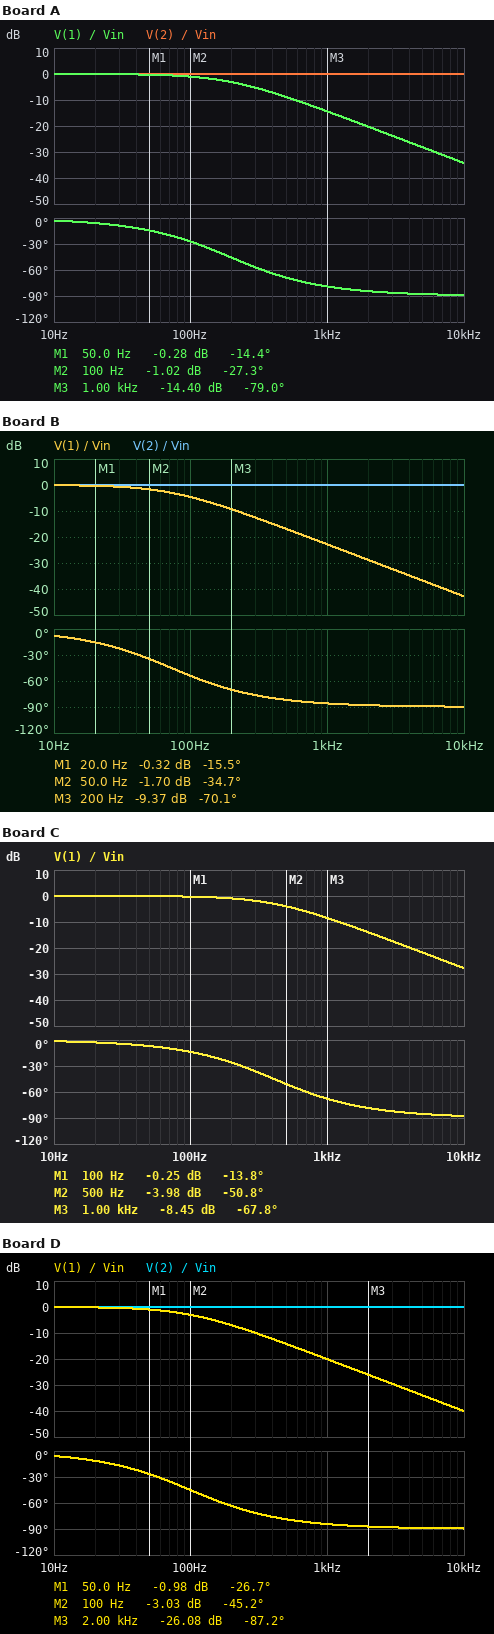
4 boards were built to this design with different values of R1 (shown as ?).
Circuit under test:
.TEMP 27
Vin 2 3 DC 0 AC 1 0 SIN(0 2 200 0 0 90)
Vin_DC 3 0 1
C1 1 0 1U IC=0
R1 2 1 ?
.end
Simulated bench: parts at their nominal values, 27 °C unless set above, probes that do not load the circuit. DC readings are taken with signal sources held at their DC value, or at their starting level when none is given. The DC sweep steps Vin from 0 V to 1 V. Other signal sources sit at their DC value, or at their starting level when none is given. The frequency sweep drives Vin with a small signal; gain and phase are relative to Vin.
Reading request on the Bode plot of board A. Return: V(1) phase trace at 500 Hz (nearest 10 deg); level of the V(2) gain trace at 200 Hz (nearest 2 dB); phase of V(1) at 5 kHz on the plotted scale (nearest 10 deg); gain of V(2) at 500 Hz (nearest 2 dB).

-70 deg
0 dB
-90 deg
0 dB
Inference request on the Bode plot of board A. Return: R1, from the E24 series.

820 Ω
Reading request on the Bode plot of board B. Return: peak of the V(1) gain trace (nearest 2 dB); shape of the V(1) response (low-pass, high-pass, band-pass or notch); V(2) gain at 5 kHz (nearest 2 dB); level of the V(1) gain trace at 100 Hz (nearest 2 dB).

0 dB
low-pass
0 dB
-4 dB
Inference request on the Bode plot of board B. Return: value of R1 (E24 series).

2.2 kΩ
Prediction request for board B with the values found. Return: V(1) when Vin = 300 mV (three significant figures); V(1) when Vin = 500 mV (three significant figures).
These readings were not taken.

1.30 V
1.50 V
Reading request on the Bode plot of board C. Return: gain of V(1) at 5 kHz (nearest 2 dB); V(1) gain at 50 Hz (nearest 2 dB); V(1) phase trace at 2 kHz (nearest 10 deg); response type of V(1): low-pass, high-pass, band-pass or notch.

-22 dB
0 dB
-80 deg
low-pass
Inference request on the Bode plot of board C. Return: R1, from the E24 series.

390 Ω
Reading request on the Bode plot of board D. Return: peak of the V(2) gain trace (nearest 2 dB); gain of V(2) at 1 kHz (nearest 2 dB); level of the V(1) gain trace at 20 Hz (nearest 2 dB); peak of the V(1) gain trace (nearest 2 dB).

0 dB
0 dB
0 dB
0 dB
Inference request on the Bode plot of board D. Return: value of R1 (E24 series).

1.6 kΩ
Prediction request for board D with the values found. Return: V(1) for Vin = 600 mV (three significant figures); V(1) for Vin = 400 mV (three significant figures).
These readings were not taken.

1.60 V
1.40 V
